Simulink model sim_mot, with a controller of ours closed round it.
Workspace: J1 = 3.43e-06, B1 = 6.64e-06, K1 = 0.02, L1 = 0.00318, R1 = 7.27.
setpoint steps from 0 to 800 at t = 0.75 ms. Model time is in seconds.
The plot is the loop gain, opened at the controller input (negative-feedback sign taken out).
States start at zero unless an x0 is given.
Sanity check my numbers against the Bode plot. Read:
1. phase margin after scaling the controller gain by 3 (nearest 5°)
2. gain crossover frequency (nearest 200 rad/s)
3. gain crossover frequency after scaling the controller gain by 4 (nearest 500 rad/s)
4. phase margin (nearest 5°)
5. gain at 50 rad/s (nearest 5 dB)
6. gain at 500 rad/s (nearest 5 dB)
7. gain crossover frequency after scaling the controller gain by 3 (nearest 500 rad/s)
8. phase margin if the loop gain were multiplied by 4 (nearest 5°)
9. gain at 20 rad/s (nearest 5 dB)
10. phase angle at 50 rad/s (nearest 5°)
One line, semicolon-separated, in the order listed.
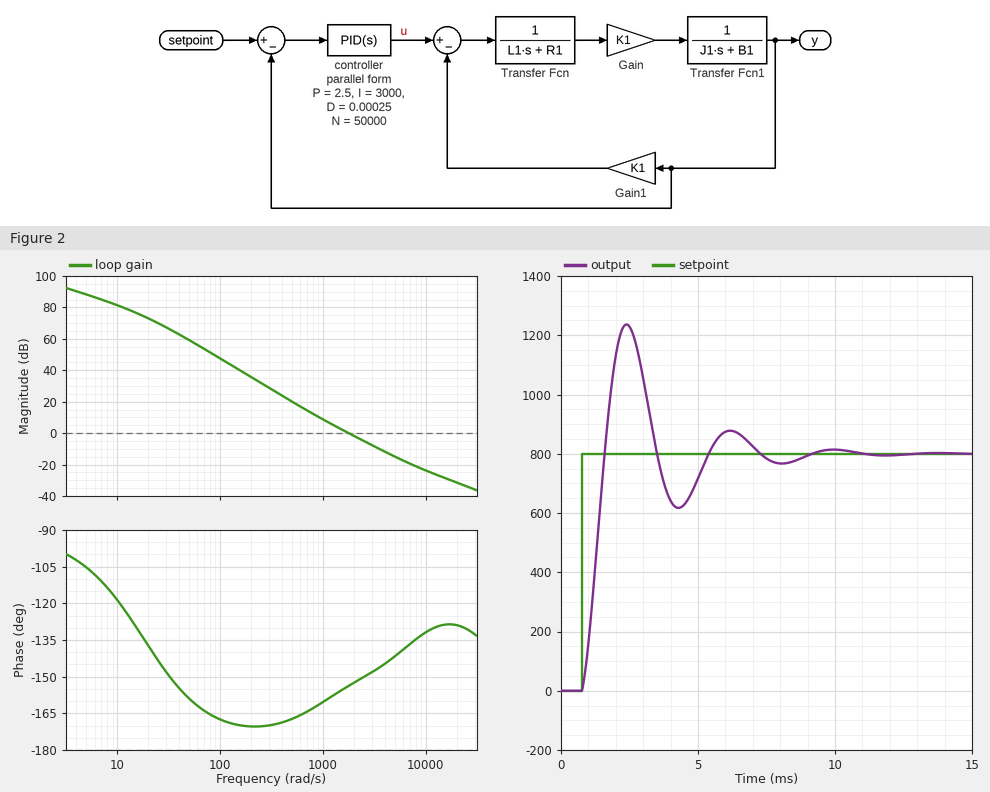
35°; 1800 rad/s; 4000 rad/s; 25°; 60 dB; 20 dB; 3500 rad/s; 35°; 75 dB; -160°
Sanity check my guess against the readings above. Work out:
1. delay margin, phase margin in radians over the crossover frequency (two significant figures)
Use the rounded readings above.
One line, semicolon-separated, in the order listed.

0.00024 s
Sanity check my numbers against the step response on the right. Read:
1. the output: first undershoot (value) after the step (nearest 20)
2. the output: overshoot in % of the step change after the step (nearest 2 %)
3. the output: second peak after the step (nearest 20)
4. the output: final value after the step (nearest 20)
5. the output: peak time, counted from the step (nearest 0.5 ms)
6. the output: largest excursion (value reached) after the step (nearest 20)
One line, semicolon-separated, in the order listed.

620; 54 %; 880; 800; 1.5 ms; 1240
